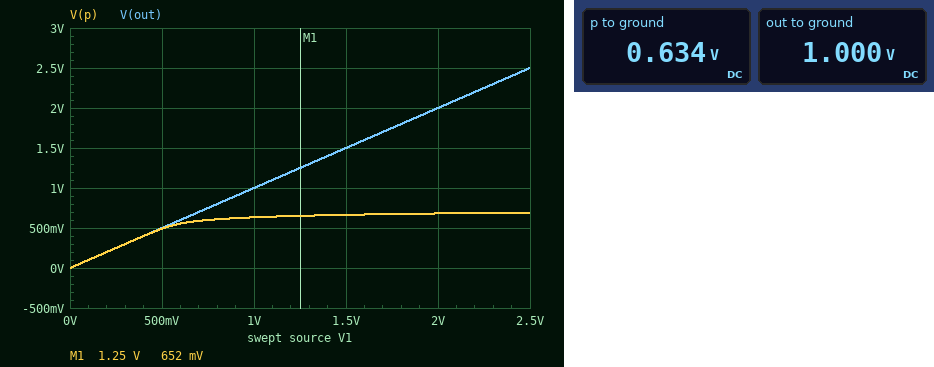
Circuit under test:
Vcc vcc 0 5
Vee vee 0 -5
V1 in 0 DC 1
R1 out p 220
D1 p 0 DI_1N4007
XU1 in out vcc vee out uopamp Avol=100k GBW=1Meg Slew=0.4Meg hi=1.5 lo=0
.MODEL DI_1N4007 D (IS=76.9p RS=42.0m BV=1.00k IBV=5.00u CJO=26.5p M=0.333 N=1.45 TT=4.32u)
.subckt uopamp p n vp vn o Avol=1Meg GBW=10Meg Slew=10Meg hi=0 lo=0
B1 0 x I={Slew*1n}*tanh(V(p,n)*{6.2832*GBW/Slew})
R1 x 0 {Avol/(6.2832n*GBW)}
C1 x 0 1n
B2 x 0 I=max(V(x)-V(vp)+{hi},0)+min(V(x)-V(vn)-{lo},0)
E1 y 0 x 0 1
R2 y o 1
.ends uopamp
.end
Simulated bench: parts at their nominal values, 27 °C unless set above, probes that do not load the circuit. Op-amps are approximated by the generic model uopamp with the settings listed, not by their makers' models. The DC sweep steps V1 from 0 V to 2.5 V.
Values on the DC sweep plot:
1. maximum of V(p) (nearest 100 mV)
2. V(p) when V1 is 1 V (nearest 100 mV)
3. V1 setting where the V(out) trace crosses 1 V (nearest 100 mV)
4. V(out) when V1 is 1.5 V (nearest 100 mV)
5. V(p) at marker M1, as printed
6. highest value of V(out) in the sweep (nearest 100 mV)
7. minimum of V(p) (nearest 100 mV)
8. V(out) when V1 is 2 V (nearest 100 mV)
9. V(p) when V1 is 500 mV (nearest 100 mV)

700 mV
600 mV
1.0 V
1.5 V
652 mV
2.5 V
0 V
2.0 V
500 mV
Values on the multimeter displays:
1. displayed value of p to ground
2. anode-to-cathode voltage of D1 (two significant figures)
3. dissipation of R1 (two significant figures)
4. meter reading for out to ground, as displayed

0.634 V
630 mV
610 µW
1.000 V
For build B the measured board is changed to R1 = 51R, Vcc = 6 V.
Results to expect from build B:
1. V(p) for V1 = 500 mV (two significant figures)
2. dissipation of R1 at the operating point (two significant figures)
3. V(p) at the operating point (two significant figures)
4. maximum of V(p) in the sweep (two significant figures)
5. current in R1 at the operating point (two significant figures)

500 mV
2.0 mW
680 mV
750 mV
6.2 mA
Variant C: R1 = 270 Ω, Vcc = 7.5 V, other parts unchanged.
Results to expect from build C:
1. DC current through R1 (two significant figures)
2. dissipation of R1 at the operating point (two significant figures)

1.4 mA
520 µW
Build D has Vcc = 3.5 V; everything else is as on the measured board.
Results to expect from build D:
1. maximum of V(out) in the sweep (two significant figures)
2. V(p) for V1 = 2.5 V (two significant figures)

2.0 V
680 mV
